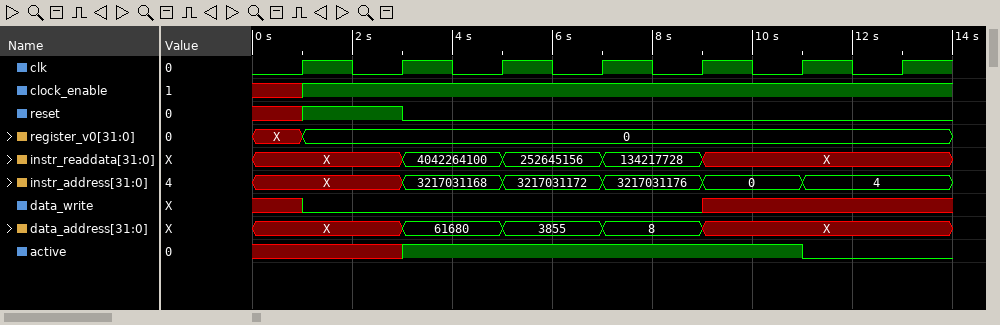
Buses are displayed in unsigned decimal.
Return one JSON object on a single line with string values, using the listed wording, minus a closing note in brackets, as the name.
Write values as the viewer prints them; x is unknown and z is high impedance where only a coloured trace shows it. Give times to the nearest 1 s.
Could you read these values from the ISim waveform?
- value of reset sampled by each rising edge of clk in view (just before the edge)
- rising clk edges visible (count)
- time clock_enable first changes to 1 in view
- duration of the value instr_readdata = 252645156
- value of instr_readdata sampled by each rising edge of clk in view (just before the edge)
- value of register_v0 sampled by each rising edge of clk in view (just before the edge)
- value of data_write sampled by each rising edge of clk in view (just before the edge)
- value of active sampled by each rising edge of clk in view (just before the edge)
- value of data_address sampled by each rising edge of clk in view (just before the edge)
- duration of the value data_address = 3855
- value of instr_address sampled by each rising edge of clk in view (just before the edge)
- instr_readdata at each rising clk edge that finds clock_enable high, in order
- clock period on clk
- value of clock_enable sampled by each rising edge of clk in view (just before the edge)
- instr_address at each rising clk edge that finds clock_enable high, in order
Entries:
{"value of reset sampled by each rising edge of clk in view": "x 1 0 0 0 0 0", "rising clk edges visible": "7", "time clock_enable first changes to 1 in view": "1 s", "duration of the value instr_readdata = 252645156": "2 s", "value of instr_readdata sampled by each rising edge of clk in view": "X, X, 4042264100, 252645156, 134217728, X, X", "value of register_v0 sampled by each rising edge of clk in view": "X, 0, 0, 0, 0, 0, 0", "value of data_write sampled by each rising edge of clk in view": "x 0 0 0 0 x x", "value of active sampled by each rising edge of clk in view": "x x 1 1 1 1 0", "value of data_address sampled by each rising edge of clk in view": "X, X, 61680, 3855, 8, X, X", "duration of the value data_address = 3855": "2 s", "value of instr_address sampled by each rising edge of clk in view": "X, X, 3217031168, 3217031172, 3217031176, 0, 4", "instr_readdata at each rising clk edge that finds clock_enable high, in order": "X, 4042264100, 252645156, 134217728, X, X", "clock period on clk": "2 s", "value of clock_enable sampled by each rising edge of clk in view": "x 1 1 1 1 1 1", "instr_address at each rising clk edge that finds clock_enable high, in order": "X, 3217031168, 3217031172, 3217031176, 0, 4"}
